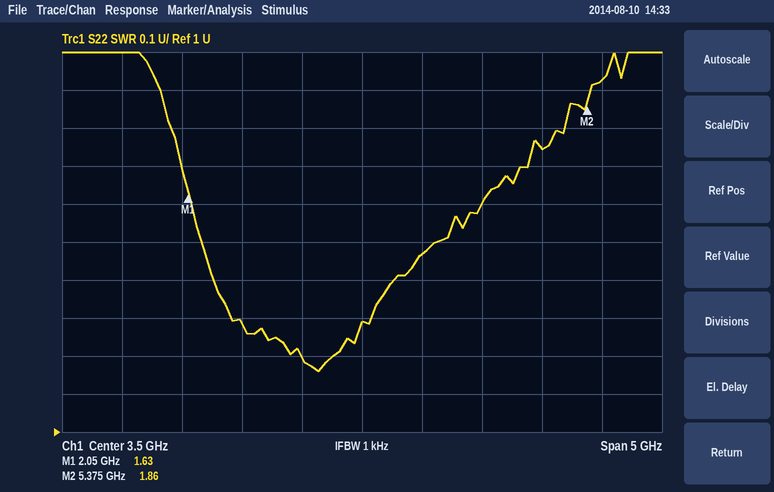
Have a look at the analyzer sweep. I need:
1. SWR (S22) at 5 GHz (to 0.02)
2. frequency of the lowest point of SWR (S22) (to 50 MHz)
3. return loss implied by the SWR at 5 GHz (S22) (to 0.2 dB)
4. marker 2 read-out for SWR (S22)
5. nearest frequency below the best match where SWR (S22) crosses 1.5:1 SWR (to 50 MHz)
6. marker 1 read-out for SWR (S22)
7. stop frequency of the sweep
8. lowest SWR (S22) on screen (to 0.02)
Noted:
1.74
3.15 GHz
11.4 dB
1.86
2.15 GHz
1.63
6 GHz
1.16
